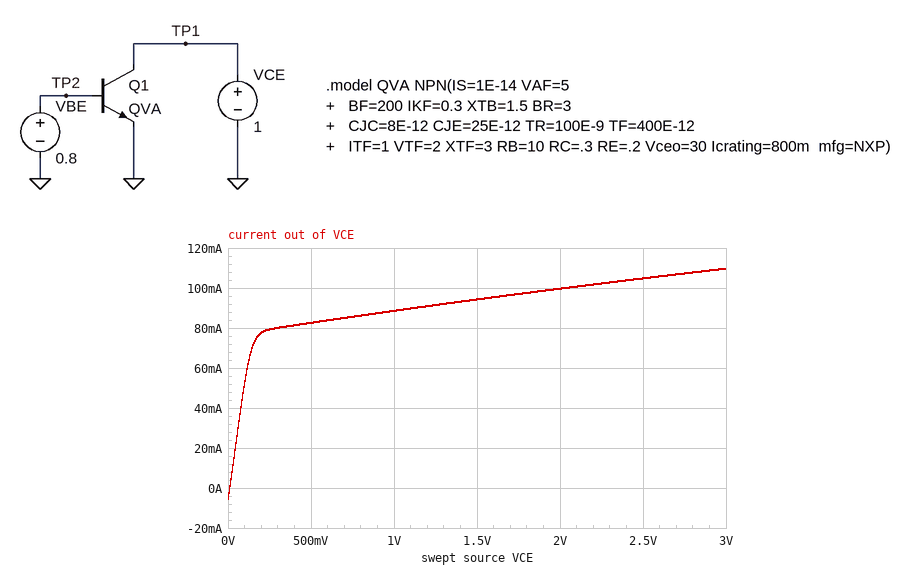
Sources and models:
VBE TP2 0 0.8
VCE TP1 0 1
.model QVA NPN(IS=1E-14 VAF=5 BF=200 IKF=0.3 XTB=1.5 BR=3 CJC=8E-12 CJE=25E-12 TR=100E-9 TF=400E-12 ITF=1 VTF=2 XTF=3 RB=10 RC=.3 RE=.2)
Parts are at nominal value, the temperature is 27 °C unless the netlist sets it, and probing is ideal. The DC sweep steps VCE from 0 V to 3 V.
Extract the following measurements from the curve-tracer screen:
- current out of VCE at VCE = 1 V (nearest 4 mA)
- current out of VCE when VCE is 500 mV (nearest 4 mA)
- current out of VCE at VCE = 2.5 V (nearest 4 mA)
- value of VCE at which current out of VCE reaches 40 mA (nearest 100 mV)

88 mA
84 mA
104 mA
100 mV
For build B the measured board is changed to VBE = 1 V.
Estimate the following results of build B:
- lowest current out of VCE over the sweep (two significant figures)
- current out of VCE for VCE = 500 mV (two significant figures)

-16 mA
450 mA
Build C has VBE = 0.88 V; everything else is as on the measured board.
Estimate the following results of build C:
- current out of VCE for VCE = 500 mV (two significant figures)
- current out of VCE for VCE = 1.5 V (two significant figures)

220 mA
250 mA
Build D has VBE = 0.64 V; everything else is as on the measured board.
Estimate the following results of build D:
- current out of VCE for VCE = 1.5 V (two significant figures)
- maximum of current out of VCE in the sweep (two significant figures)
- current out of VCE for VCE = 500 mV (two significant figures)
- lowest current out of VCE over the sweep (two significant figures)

650 µA
810 µA
540 µA
-170 µA
